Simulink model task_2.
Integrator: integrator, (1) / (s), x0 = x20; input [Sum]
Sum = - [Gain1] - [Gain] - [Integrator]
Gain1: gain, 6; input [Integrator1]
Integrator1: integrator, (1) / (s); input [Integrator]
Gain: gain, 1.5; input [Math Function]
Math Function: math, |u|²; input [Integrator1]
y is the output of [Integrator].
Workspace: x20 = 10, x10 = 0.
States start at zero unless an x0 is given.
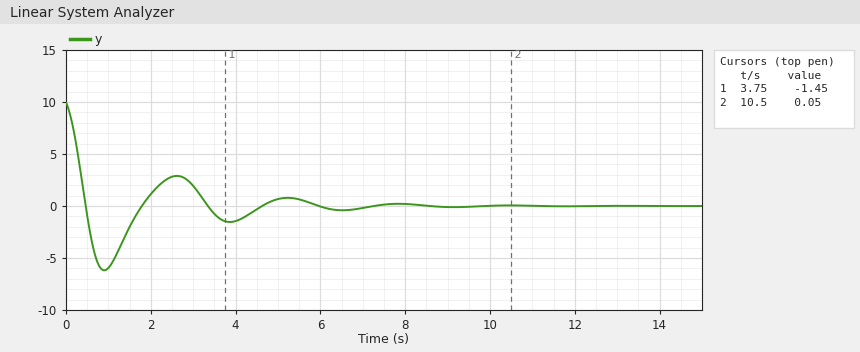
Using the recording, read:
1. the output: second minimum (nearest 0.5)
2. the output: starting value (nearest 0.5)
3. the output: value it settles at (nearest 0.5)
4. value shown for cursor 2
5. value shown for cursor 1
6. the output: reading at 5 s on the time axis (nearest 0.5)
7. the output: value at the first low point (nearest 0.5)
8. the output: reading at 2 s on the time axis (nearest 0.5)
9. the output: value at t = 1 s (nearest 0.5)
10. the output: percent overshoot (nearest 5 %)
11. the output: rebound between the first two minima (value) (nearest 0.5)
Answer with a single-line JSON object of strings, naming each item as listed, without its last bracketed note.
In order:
{"the output: second minimum": "-1.5", "the output: starting value": "10.0", "the output: value it settles at": "0.0", "value shown for cursor 2": "0.05", "value shown for cursor 1": "-1.45", "the output: reading at 5 s on the time axis": "0.5", "the output: value at the first low point": "-6.0", "the output: reading at 2 s on the time axis": "1.0", "the output: value at t = 1 s": "-6.0", "the output: percent overshoot": "60 %", "the output: rebound between the first two minima (value)": "3.0"}
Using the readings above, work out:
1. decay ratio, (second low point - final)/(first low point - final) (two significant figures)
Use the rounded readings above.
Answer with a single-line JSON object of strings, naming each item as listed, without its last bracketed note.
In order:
{"decay ratio, (second low point - final)/(first low point - final)": "0.25"}
